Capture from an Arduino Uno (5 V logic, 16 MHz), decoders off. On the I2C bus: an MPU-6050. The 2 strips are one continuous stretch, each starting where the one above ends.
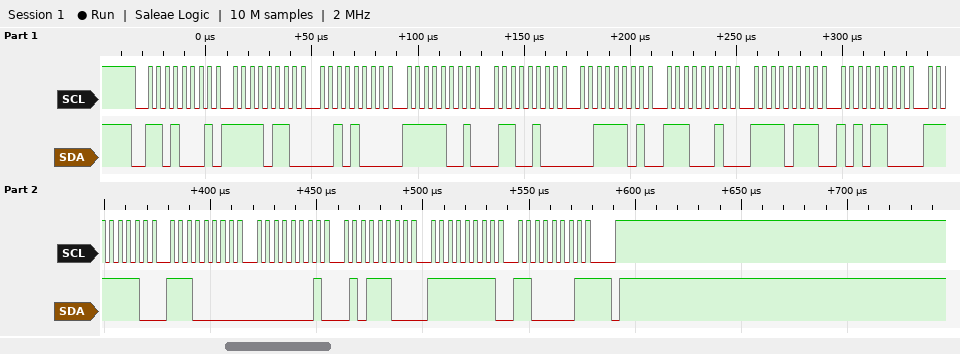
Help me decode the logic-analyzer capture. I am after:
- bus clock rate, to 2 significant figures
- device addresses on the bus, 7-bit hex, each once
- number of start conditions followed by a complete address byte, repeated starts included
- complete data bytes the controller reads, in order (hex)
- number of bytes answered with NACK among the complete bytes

250 kHz
0x68
1
F6 28 F9 64 3D E2 F7 AC FE E0 01 5C FF C1
1
